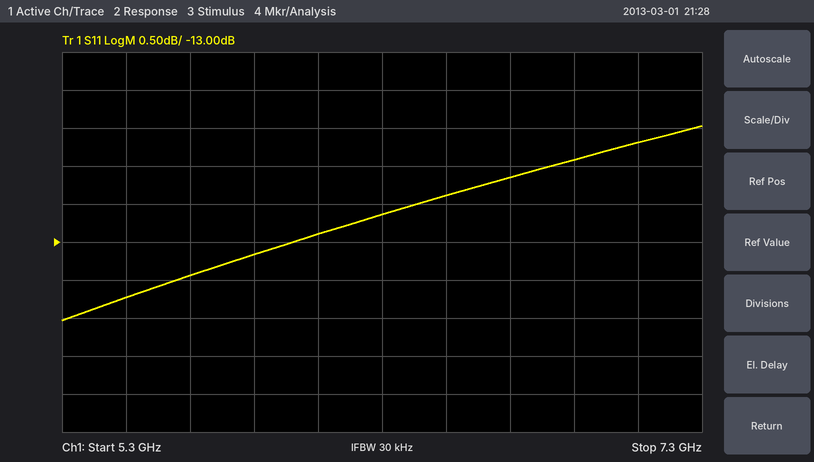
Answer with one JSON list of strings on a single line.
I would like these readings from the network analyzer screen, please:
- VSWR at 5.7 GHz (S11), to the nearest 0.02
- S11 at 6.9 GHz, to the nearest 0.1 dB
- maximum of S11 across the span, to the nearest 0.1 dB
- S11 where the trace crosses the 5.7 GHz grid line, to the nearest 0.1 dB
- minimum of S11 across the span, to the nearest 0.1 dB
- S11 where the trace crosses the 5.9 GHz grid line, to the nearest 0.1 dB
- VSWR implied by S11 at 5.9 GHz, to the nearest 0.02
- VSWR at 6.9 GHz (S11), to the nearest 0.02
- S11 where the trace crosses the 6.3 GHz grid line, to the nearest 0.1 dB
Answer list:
["1.54", "-11.9 dB", "-11.5 dB", "-13.4 dB", "-14.0 dB", "-13.2 dB", "1.56", "1.68", "-12.6 dB"]
